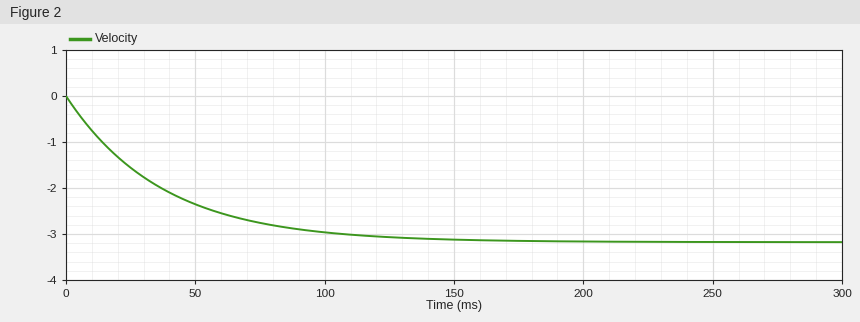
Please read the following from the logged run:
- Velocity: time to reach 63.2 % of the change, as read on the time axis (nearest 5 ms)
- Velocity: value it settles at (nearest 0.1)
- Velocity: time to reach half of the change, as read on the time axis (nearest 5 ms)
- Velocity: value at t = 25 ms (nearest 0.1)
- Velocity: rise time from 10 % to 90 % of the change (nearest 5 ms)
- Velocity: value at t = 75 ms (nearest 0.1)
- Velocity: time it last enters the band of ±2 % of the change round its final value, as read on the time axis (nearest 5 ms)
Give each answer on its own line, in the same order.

35 ms
-3.2
25 ms
-1.6
80 ms
-2.8
145 ms
